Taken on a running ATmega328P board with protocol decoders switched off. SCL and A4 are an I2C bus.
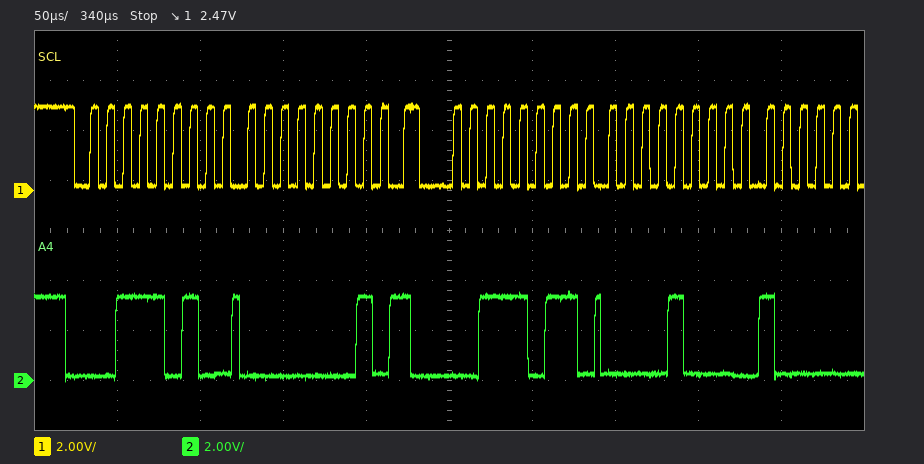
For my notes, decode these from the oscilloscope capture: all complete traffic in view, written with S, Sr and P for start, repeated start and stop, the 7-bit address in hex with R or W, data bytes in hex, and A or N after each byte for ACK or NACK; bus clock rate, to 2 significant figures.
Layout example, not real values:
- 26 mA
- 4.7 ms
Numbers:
- S 1DW A 01 A Sr 1DR A 08 A
- 100 kHz
